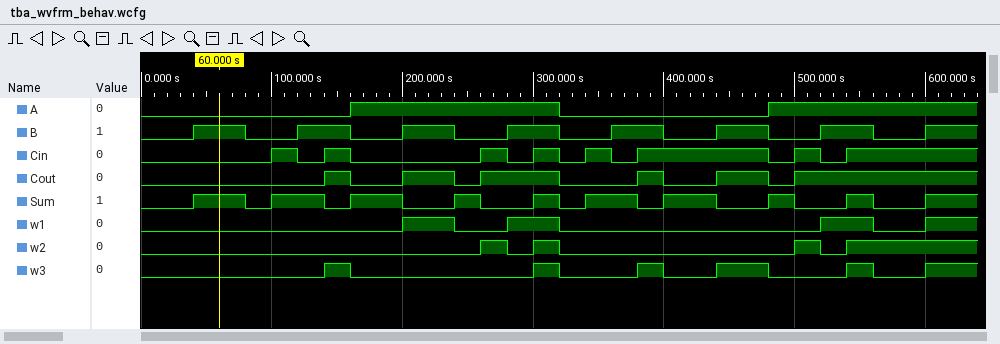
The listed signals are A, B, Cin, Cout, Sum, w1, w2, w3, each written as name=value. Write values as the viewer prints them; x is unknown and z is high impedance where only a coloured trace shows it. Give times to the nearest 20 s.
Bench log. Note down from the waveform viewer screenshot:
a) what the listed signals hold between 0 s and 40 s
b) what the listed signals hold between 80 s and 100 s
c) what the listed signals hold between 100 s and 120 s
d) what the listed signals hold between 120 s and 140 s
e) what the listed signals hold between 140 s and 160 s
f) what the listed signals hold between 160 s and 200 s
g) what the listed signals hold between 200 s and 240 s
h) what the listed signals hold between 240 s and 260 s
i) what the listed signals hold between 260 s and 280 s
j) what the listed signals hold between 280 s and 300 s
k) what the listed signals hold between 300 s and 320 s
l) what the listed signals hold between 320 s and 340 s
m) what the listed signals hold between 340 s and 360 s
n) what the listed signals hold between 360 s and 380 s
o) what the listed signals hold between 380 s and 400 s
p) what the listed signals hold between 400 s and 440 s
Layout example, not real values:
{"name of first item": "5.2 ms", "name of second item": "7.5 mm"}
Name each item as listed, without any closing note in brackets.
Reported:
{"what the listed signals hold between 0 s and 40 s": "A=0, B=0, Cin=0, Cout=0, Sum=0, w1=0, w2=0, w3=0", "what the listed signals hold between 80 s and 100 s": "A=0, B=0, Cin=0, Cout=0, Sum=0, w1=0, w2=0, w3=0", "what the listed signals hold between 100 s and 120 s": "A=0, B=0, Cin=1, Cout=0, Sum=1, w1=0, w2=0, w3=0", "what the listed signals hold between 120 s and 140 s": "A=0, B=1, Cin=0, Cout=0, Sum=1, w1=0, w2=0, w3=0", "what the listed signals hold between 140 s and 160 s": "A=0, B=1, Cin=1, Cout=1, Sum=0, w1=0, w2=0, w3=1", "what the listed signals hold between 160 s and 200 s": "A=1, B=0, Cin=0, Cout=0, Sum=1, w1=0, w2=0, w3=0", "what the listed signals hold between 200 s and 240 s": "A=1, B=1, Cin=0, Cout=1, Sum=0, w1=1, w2=0, w3=0", "what the listed signals hold between 240 s and 260 s": "A=1, B=0, Cin=0, Cout=0, Sum=1, w1=0, w2=0, w3=0", "what the listed signals hold between 260 s and 280 s": "A=1, B=0, Cin=1, Cout=1, Sum=0, w1=0, w2=1, w3=0", "what the listed signals hold between 280 s and 300 s": "A=1, B=1, Cin=0, Cout=1, Sum=0, w1=1, w2=0, w3=0", "what the listed signals hold between 300 s and 320 s": "A=1, B=1, Cin=1, Cout=1, Sum=1, w1=1, w2=1, w3=1", "what the listed signals hold between 320 s and 340 s": "A=0, B=0, Cin=0, Cout=0, Sum=0, w1=0, w2=0, w3=0", "what the listed signals hold between 340 s and 360 s": "A=0, B=0, Cin=1, Cout=0, Sum=1, w1=0, w2=0, w3=0", "what the listed signals hold between 360 s and 380 s": "A=0, B=1, Cin=0, Cout=0, Sum=1, w1=0, w2=0, w3=0", "what the listed signals hold between 380 s and 400 s": "A=0, B=1, Cin=1, Cout=1, Sum=0, w1=0, w2=0, w3=1", "what the listed signals hold between 400 s and 440 s": "A=0, B=0, Cin=1, Cout=0, Sum=1, w1=0, w2=0, w3=0"}
